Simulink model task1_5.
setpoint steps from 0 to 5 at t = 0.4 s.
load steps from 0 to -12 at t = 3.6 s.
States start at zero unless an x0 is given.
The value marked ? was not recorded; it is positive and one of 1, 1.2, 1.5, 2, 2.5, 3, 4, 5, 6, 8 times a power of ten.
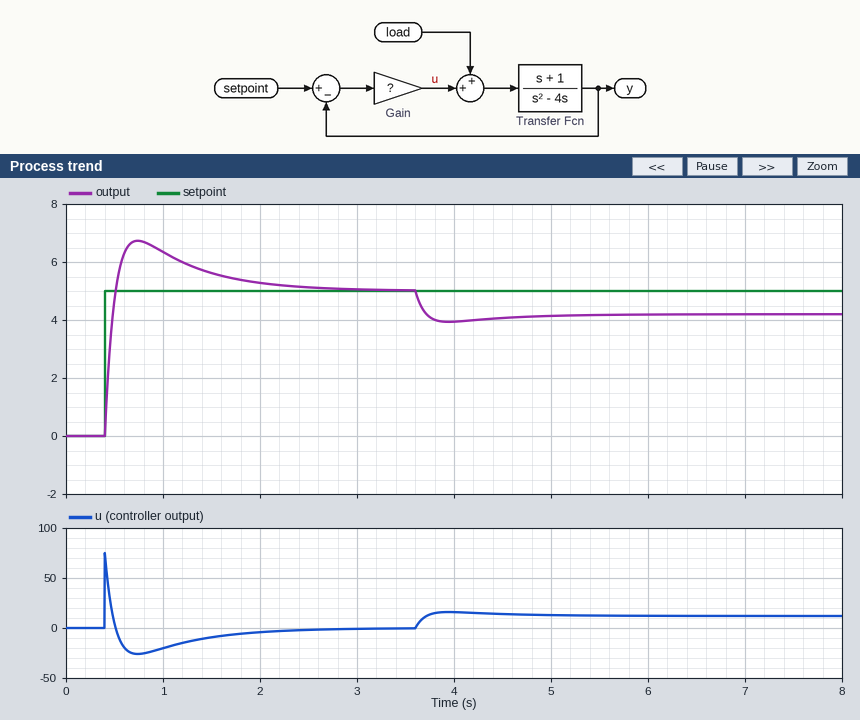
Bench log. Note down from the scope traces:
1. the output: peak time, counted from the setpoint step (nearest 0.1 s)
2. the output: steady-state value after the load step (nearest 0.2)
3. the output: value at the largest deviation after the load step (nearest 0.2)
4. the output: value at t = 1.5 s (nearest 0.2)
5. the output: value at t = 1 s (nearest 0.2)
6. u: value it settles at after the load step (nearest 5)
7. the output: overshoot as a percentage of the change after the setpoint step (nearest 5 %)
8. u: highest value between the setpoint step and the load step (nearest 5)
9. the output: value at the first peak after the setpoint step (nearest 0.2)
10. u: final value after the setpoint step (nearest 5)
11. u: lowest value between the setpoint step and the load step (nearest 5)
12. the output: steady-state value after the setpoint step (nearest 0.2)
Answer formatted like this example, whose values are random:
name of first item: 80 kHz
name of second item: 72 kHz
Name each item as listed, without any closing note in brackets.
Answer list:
the output: peak time, counted from the setpoint step: 0.3 s
the output: steady-state value after the load step: 4.2
the output: value at the largest deviation after the load step: 4.0
the output: value at t = 1.5 s: 5.6
the output: value at t = 1 s: 6.4
u: value it settles at after the load step: 10
the output: overshoot as a percentage of the change after the setpoint step: 35 %
u: highest value between the setpoint step and the load step: 75
the output: value at the first peak after the setpoint step: 6.8
u: final value after the setpoint step: 0
u: lowest value between the setpoint step and the load step: -25
the output: steady-state value after the setpoint step: 5.0
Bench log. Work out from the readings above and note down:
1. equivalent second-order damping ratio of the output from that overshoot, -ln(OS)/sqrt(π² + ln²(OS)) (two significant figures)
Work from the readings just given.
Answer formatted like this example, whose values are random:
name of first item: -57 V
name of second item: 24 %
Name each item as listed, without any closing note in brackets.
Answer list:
equivalent second-order damping ratio of the output from that overshoot, -ln(OS)/sqrt(π² + ln²(OS)): 0.32
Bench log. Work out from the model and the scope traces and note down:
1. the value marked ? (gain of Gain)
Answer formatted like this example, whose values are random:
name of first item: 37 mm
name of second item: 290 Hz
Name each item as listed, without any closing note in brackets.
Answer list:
the value marked ?: 15
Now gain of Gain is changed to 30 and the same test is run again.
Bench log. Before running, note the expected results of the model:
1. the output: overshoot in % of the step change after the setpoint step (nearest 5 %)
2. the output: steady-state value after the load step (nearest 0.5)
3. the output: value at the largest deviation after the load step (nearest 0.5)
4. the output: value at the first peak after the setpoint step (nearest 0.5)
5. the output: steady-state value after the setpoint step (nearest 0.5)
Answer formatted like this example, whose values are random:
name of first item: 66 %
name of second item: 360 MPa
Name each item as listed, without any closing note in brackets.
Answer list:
the output: overshoot in % of the step change after the setpoint step: 15 %
the output: steady-state value after the load step: 4.5
the output: value at the largest deviation after the load step: 4.5
the output: value at the first peak after the setpoint step: 6.0
the output: steady-state value after the setpoint step: 5.0
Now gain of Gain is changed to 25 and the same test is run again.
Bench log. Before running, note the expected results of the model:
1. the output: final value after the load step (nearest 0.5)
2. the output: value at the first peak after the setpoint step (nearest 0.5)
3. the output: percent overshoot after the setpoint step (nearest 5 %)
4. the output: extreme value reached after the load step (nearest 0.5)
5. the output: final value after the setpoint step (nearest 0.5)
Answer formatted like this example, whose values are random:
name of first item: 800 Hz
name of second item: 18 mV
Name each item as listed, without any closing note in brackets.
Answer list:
the output: final value after the load step: 4.5
the output: value at the first peak after the setpoint step: 6.0
the output: percent overshoot after the setpoint step: 20 %
the output: extreme value reached after the load step: 4.5
the output: final value after the setpoint step: 5.0
